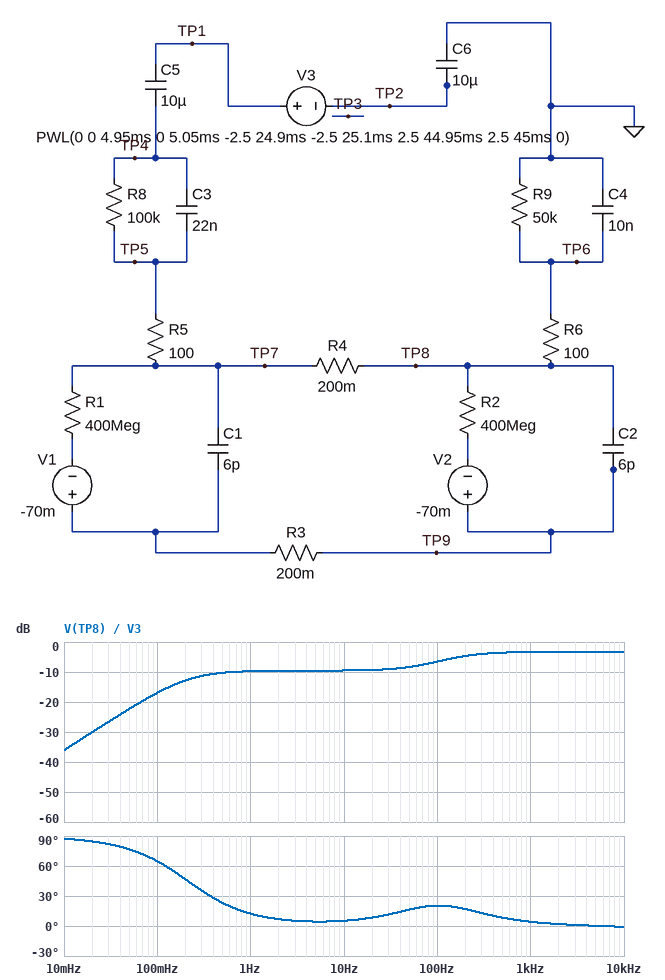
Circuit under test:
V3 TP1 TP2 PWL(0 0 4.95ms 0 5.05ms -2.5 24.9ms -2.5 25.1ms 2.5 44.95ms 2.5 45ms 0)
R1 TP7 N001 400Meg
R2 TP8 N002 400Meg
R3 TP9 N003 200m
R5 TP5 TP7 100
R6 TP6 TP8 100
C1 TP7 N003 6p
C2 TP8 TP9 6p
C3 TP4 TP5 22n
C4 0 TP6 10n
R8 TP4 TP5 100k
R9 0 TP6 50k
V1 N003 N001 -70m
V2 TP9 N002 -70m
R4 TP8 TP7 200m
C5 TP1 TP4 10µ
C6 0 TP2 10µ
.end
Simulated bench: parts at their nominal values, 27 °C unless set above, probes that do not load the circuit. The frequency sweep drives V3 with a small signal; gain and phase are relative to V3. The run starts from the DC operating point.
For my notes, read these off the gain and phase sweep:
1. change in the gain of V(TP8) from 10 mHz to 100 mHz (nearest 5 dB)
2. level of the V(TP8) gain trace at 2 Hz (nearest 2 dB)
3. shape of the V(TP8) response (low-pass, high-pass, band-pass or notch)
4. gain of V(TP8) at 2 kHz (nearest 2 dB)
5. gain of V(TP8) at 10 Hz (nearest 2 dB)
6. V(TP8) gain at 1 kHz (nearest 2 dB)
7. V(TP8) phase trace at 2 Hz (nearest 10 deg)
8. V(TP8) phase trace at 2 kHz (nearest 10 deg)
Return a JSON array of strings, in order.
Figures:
["20 dB", "-10 dB", "high-pass", "-4 dB", "-10 dB", "-4 dB", "10 deg", "0 deg"]
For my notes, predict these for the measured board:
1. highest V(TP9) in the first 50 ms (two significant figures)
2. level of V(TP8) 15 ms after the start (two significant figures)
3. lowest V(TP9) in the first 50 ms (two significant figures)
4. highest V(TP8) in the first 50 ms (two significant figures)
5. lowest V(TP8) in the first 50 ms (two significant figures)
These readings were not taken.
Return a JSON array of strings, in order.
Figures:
["2.4 V", "-820 mV", "-1.7 V", "2.5 V", "-1.7 V"]
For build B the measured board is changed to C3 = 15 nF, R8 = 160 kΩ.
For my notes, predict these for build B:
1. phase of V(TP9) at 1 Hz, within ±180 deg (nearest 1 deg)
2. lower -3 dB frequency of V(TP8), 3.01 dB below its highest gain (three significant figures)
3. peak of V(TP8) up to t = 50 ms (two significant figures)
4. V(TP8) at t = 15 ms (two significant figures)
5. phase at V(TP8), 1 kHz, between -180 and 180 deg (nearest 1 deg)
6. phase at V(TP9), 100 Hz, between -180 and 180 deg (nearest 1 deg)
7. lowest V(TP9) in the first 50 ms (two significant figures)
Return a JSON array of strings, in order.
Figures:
["9 deg", "138 Hz", "2.2 V", "-590 mV", "6 deg", "26 deg", "-1.5 V"]
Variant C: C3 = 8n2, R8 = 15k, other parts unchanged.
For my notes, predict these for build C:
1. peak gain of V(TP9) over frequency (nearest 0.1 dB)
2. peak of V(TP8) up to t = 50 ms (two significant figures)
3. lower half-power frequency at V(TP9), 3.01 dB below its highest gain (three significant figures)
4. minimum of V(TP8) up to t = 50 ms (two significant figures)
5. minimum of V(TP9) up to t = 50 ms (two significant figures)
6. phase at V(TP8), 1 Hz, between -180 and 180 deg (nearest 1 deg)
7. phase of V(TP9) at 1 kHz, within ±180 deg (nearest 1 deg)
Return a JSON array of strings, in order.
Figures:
["-2.3 dB", "2.0 V", "487 mHz", "-1.9 V", "-2.0 V", "26 deg", "-15 deg"]
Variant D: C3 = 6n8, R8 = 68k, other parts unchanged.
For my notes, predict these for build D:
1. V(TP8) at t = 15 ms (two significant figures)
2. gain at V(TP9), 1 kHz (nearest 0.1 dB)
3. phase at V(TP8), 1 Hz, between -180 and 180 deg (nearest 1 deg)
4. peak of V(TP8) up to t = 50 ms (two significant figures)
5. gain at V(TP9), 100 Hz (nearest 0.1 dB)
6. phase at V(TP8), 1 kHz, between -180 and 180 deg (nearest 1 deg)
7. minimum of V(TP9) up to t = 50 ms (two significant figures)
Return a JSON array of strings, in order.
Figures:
["-1.0 V", "-7.8 dB", "15 deg", "1.1 V", "-7.5 dB", "-1 deg", "-1.1 V"]
